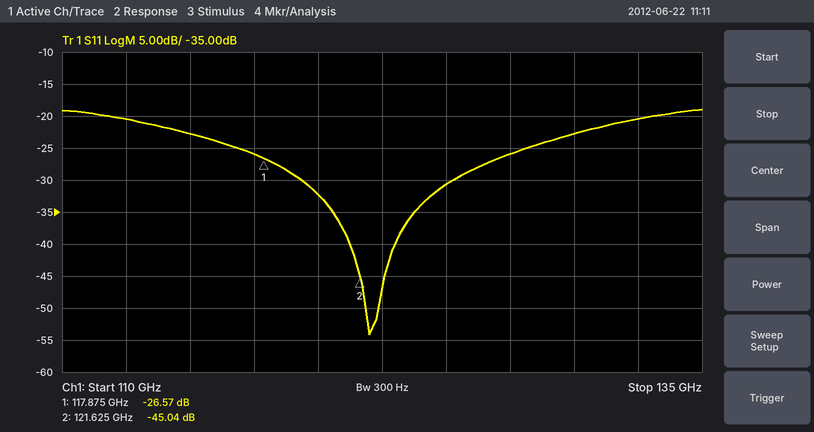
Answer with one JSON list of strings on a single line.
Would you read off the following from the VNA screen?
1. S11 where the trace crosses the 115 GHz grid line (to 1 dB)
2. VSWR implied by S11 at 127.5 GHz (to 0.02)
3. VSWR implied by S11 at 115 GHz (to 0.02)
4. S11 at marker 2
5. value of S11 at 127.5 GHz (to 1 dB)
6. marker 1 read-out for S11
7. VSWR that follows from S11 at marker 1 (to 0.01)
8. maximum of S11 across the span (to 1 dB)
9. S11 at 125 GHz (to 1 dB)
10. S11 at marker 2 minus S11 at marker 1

["-23 dB", "1.10", "1.16", "-45.04 dB", "-26 dB", "-26.57 dB", "1.10", "-19 dB", "-31 dB", "-18.47 dB"]
